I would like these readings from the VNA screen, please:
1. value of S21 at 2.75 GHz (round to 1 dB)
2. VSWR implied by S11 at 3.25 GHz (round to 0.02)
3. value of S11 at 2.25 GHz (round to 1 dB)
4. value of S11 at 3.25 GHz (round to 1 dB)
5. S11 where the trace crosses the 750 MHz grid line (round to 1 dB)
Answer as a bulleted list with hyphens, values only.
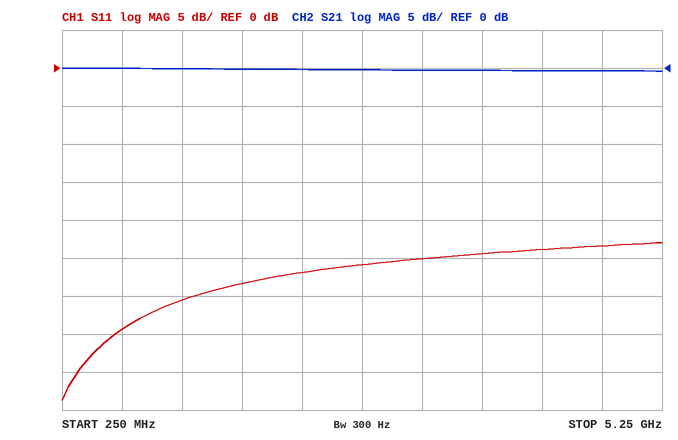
- 0 dB
- 1.12
- -27 dB
- -25 dB
- -34 dB
